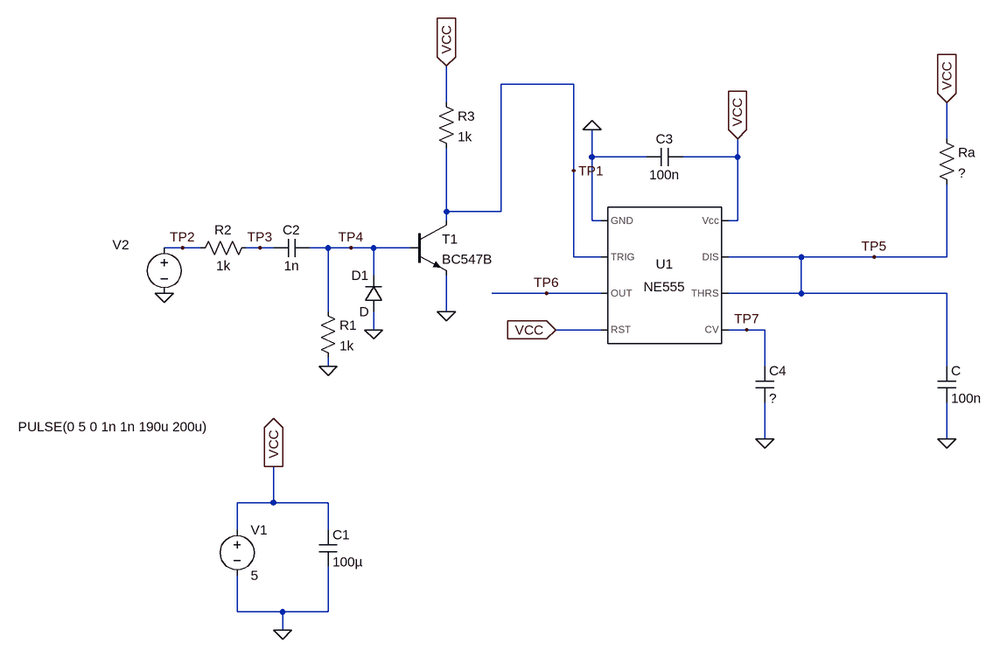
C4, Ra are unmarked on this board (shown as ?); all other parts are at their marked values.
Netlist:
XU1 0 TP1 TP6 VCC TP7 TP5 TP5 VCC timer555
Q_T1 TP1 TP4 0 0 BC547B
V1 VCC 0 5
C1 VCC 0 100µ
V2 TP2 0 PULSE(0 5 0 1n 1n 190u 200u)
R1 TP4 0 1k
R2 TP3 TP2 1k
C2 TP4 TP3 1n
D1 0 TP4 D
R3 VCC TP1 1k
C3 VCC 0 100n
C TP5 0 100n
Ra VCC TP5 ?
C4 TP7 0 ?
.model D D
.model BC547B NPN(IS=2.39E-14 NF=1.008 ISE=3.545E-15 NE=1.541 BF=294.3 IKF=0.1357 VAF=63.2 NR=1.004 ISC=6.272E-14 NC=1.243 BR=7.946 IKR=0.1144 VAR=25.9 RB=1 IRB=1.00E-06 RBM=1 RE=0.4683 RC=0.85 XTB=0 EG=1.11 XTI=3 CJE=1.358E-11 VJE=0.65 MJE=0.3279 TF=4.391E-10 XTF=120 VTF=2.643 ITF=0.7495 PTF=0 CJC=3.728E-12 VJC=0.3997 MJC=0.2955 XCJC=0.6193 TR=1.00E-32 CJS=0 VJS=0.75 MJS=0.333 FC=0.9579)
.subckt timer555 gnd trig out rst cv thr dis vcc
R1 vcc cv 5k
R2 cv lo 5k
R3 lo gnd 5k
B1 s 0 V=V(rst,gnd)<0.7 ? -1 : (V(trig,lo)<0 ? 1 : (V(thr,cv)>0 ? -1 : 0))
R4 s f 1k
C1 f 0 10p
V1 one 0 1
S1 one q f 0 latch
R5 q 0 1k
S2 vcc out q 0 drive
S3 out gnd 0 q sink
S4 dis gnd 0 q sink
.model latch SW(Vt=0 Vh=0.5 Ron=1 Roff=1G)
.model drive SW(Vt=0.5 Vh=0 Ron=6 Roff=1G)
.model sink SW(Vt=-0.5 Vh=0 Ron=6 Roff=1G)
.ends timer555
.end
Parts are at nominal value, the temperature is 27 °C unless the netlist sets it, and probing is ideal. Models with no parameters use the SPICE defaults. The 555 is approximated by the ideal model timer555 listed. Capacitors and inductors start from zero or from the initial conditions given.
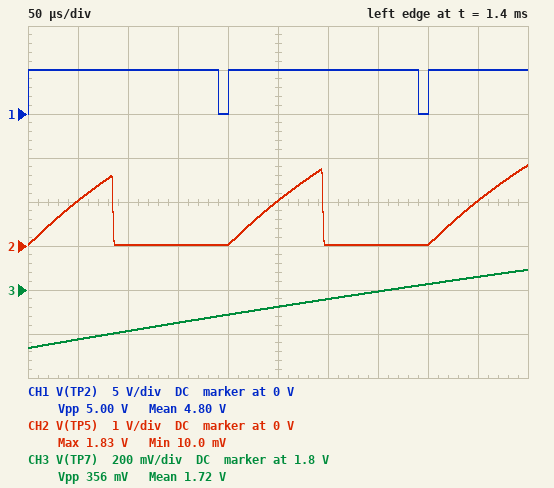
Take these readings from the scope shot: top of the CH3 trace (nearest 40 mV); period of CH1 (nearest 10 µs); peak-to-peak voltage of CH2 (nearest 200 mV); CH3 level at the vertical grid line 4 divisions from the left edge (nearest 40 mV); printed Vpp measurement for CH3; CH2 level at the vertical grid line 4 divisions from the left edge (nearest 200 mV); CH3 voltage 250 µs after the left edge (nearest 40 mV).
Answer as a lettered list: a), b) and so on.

a) 1.88 V
b) 200 µs
c) 1.8 V
d) 1.68 V
e) 356 mV
f) 0 V
g) 1.72 V
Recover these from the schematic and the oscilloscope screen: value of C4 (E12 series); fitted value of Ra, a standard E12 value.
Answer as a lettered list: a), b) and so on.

a) 680 nF
b) 2.2 kΩ
